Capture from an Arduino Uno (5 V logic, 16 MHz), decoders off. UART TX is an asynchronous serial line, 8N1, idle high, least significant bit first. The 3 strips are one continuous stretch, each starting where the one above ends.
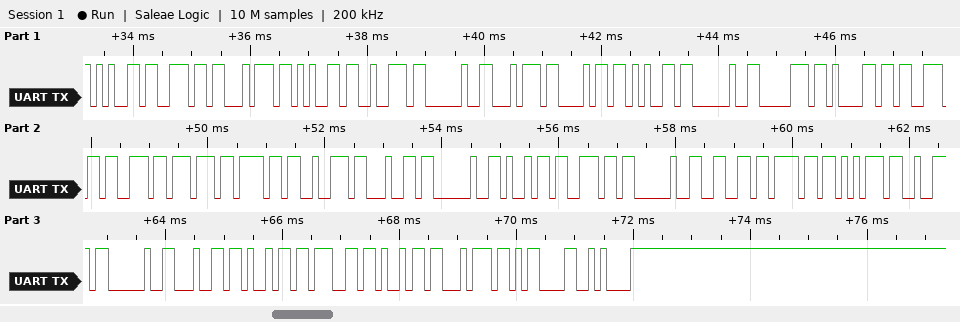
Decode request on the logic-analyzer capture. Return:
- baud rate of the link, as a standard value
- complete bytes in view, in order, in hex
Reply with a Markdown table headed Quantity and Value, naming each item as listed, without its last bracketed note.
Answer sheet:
| Quantity | Value |
|---|---|
| baud rate of the link, as a standard value | 9600 baud |
| complete bytes in view, in order, in hex | 65 6E 74 65 72 20 74 68 65 20 70 61 73 73 77 6F 72 64 20 69 6E 20 66 6F 75 72 20 64 69 67 69 74 0D 0A |
